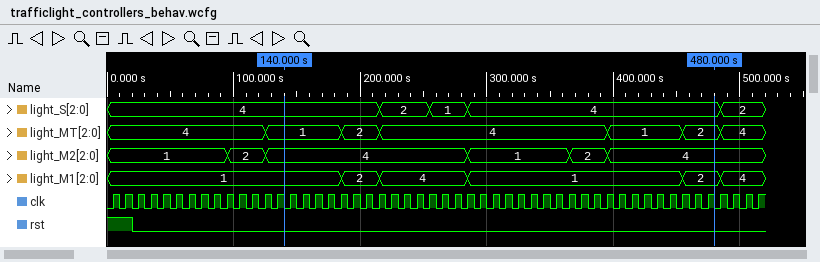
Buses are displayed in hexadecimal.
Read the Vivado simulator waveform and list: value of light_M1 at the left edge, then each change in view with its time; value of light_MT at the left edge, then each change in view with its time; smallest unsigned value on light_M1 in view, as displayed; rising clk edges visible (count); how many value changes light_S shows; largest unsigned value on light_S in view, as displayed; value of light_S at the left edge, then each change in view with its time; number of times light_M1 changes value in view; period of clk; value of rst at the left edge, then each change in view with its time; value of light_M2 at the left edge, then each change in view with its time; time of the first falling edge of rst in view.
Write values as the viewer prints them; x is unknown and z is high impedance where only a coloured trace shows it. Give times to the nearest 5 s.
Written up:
1, 2 at 185 s, 4 at 215 s, 1 at 285 s, 2 at 455 s, 4 at 485 s
4, 1 at 125 s, 2 at 185 s, 4 at 215 s, 1 at 395 s, 2 at 455 s, 4 at 485 s
1
52
4
4
4, 2 at 215 s, 1 at 255 s, 4 at 285 s, 2 at 485 s
5
10 s
1, 0 at 20 s
1, 2 at 95 s, 4 at 125 s, 1 at 285 s, 2 at 365 s, 4 at 395 s
20 s
